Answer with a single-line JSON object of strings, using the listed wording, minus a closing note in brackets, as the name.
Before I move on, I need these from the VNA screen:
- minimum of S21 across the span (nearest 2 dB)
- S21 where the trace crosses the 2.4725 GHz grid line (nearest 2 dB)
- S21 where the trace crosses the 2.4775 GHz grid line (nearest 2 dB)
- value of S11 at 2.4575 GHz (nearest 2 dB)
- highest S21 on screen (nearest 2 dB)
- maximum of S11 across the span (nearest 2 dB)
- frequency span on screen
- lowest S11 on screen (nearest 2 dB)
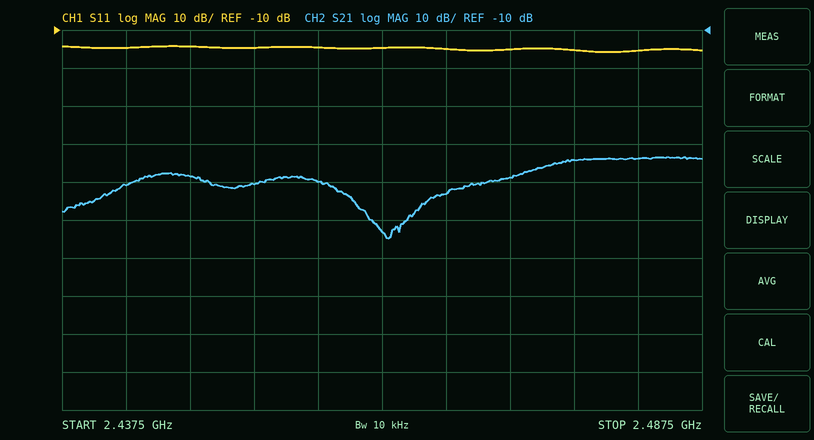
{"minimum of S21 across the span": "-64 dB", "S21 where the trace crosses the 2.4725 GHz grid line": "-48 dB", "S21 where the trace crosses the 2.4775 GHz grid line": "-44 dB", "value of S11 at 2.4575 GHz": "-14 dB", "highest S21 on screen": "-44 dB", "maximum of S11 across the span": "-14 dB", "frequency span on screen": "50 MHz", "lowest S11 on screen": "-16 dB"}
